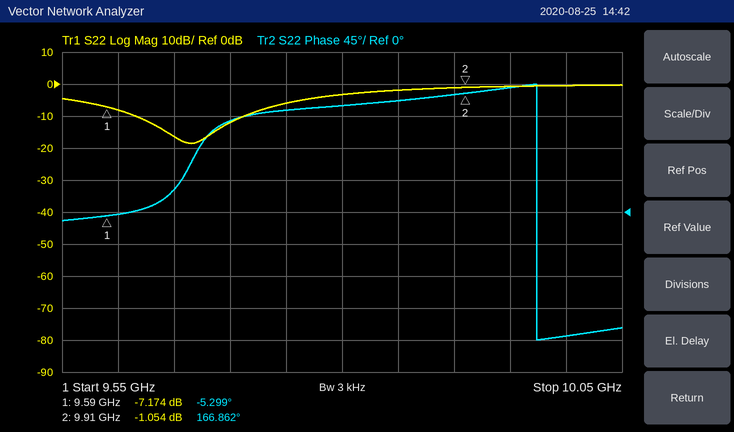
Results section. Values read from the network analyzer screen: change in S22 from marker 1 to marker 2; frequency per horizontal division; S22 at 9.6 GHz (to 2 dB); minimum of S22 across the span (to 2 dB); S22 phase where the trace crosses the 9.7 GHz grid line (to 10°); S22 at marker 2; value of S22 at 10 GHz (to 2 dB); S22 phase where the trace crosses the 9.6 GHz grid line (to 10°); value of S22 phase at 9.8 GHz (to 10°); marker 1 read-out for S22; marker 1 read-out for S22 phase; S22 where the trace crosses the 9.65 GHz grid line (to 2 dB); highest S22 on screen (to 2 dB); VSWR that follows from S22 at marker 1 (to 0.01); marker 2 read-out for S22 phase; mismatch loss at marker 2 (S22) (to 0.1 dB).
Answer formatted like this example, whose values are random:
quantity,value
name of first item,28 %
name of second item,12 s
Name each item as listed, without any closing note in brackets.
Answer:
quantity,value
change in S22 from marker 1 to marker 2,6.120 dB
frequency per horizontal division,50 MHz
S22 at 9.6 GHz,-8 dB
minimum of S22 across the span,-18 dB
S22 phase where the trace crosses the 9.7 GHz grid line,130°
S22 at marker 2,-1.054 dB
value of S22 at 10 GHz,0 dB
S22 phase where the trace crosses the 9.6 GHz grid line,0°
value of S22 phase at 9.8 GHz,150°
marker 1 read-out for S22,-7.174 dB
marker 1 read-out for S22 phase,-5.299°
S22 where the trace crosses the 9.65 GHz grid line,-16 dB
highest S22 on screen,0 dB
VSWR that follows from S22 at marker 1,2.56
marker 2 read-out for S22 phase,166.862°
mismatch loss at marker 2 (S22),6.7 dB
